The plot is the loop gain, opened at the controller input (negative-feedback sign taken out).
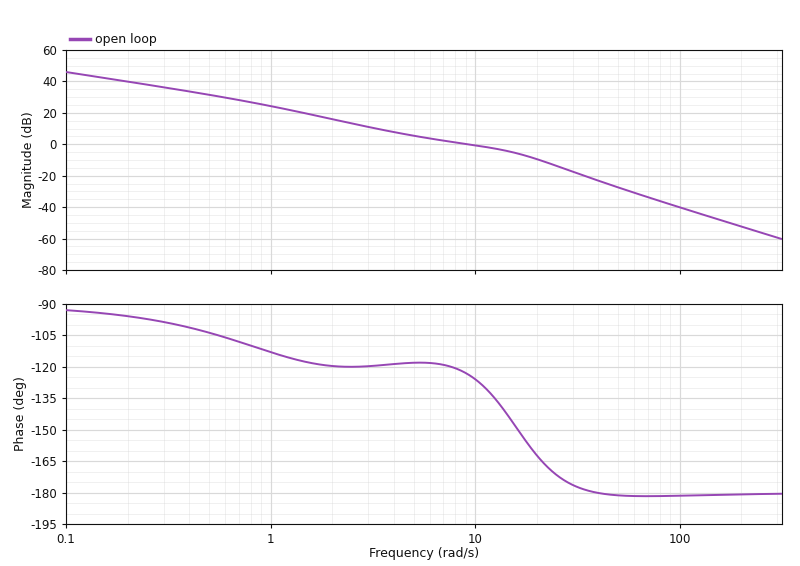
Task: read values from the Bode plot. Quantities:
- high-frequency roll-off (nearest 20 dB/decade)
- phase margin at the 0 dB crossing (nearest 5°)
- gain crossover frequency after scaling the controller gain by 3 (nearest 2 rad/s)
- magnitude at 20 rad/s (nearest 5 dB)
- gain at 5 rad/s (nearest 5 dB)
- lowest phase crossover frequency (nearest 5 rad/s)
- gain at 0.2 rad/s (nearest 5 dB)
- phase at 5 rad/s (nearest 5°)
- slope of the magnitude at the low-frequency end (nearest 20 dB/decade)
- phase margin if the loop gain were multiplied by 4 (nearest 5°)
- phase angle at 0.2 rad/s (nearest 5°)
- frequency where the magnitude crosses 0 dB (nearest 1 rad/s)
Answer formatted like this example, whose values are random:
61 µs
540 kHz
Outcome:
-40 dB/decade
55°
20 rad/s
-10 dB
5 dB
40 rad/s
40 dB
-120°
-20 dB/decade
10°
-95°
9 rad/s
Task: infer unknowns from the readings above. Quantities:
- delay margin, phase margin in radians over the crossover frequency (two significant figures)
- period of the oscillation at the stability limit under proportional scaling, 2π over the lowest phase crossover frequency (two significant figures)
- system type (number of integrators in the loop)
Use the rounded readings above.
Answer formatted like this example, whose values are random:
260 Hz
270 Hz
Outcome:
0.11 s
0.16 s
1
